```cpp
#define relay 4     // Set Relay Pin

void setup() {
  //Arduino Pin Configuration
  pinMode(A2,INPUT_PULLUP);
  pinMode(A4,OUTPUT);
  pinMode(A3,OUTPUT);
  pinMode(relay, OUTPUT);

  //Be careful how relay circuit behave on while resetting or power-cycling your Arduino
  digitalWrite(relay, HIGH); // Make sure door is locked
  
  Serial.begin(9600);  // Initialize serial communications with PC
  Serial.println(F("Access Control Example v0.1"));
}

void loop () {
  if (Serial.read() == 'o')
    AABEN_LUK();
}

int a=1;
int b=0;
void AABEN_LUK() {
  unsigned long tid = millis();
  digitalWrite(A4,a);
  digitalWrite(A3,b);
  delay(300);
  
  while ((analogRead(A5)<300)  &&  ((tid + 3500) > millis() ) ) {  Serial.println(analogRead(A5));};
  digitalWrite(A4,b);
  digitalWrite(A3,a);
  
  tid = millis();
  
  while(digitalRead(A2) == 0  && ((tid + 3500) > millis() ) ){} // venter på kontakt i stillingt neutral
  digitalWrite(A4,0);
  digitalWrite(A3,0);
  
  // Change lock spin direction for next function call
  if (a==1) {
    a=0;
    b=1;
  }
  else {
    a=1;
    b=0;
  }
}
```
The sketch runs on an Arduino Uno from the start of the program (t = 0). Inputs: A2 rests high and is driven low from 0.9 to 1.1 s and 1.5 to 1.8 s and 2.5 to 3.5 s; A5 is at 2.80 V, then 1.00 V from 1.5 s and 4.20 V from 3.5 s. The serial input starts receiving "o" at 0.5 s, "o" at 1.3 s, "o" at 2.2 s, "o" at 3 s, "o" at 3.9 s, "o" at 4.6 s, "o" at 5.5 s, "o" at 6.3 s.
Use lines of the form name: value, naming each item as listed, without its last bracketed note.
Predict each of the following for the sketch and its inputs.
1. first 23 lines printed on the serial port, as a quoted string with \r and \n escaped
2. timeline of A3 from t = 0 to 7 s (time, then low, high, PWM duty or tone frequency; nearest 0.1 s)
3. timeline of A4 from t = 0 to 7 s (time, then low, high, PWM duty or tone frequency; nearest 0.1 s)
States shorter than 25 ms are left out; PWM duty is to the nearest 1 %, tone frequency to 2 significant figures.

first 23 lines printed on the serial port, as a quoted string with \r and \n escaped: "Access Control Example v0.1\r\n204\r\n204\r\n204\r\n204\r\n204\r\n204\r\n204\r\n204\r\n204\r\n204\r\n204\r\n204\r\n204\r\n204\r\n204\r\n204\r\n204\r\n204\r\n204\r\n204\r\n204\r\n204\r\n"
timeline of A3 from t = 0 to 7 s: 0 s low; 1.3 s high; 3.5 s low; 3.8 s high; 4.1 s low; 4.6 s high; 4.9 s low; 6.3 s high; 6.6 s low
timeline of A4 from t = 0 to 7 s: 0 s low; 0.5 s high; 0.8 s low; 3.5 s high; 3.8 s low; 4.1 s high; 4.4 s low; 5.5 s high; 5.8 s low
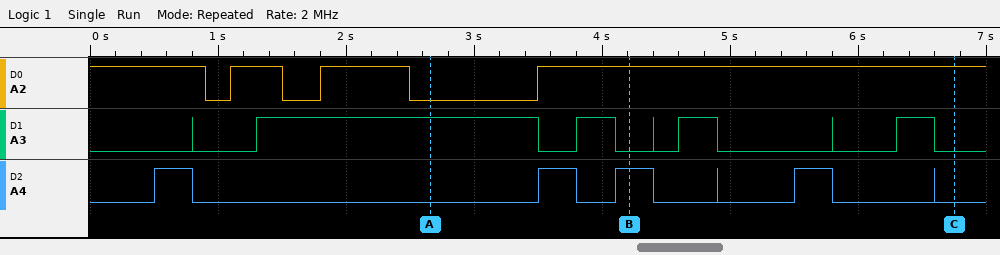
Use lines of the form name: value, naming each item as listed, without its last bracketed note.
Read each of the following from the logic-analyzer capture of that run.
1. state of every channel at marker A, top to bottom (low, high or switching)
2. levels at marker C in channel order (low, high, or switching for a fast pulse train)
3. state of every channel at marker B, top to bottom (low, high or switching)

state of every channel at marker A, top to bottom: A2 low, A3 high, A4 low
levels at marker C in channel order: A2 high, A3 low, A4 low
state of every channel at marker B, top to bottom: A2 high, A3 low, A4 high
